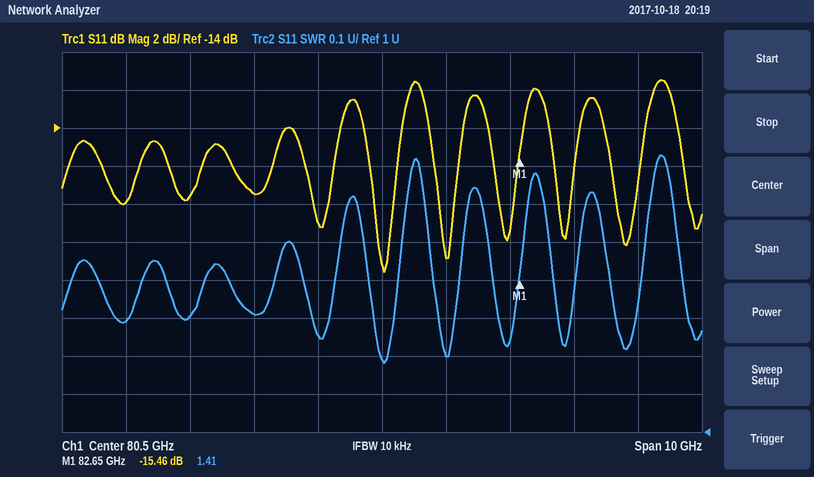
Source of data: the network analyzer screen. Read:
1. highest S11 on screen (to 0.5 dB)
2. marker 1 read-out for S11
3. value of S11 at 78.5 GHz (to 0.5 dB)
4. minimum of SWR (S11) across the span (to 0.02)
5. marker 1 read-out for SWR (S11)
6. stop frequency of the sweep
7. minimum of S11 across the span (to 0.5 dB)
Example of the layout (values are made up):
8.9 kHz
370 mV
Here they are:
-11.5 dB
-15.46 dB
-17.5 dB
1.18
1.41
85.5 GHz
-21.5 dB
